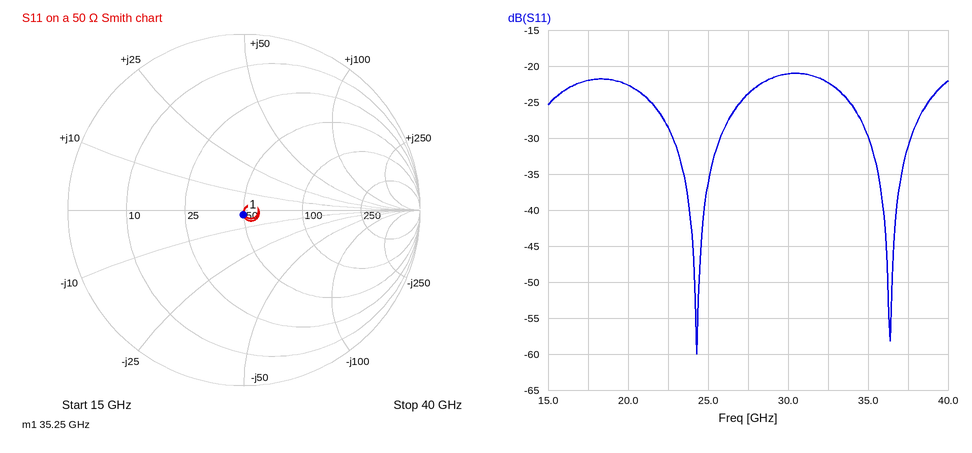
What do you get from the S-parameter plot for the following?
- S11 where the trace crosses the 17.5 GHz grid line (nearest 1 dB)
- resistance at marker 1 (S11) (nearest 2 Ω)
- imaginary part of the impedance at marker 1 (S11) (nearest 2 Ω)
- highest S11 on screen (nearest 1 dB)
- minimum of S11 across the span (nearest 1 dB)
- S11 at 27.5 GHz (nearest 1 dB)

-22 dB
50 Ω
-2 Ω
-21 dB
-60 dB
-24 dB
